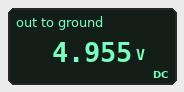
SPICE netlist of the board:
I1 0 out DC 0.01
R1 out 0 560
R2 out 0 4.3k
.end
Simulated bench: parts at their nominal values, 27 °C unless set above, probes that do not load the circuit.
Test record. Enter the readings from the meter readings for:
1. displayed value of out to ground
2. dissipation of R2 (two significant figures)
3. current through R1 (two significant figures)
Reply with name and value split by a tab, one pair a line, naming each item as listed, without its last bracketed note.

displayed value of out to ground	4.955 V
dissipation of R2	5.7 mW
current through R1	8.8 mA
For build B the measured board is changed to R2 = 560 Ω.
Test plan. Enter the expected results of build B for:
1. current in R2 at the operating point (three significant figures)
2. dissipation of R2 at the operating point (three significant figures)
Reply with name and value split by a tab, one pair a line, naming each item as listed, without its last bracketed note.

current in R2 at the operating point	5.00 mA
dissipation of R2 at the operating point	14.0 mW
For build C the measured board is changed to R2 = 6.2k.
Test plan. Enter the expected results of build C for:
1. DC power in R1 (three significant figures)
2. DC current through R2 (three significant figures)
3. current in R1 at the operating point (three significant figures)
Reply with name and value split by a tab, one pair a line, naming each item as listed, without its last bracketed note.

DC power in R1	47.1 mW
DC current through R2	828 µA
current in R1 at the operating point	9.17 mA
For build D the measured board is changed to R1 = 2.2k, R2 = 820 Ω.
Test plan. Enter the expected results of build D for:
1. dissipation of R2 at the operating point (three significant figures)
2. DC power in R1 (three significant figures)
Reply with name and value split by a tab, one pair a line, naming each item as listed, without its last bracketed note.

dissipation of R2 at the operating point	43.5 mW
DC power in R1	16.2 mW
